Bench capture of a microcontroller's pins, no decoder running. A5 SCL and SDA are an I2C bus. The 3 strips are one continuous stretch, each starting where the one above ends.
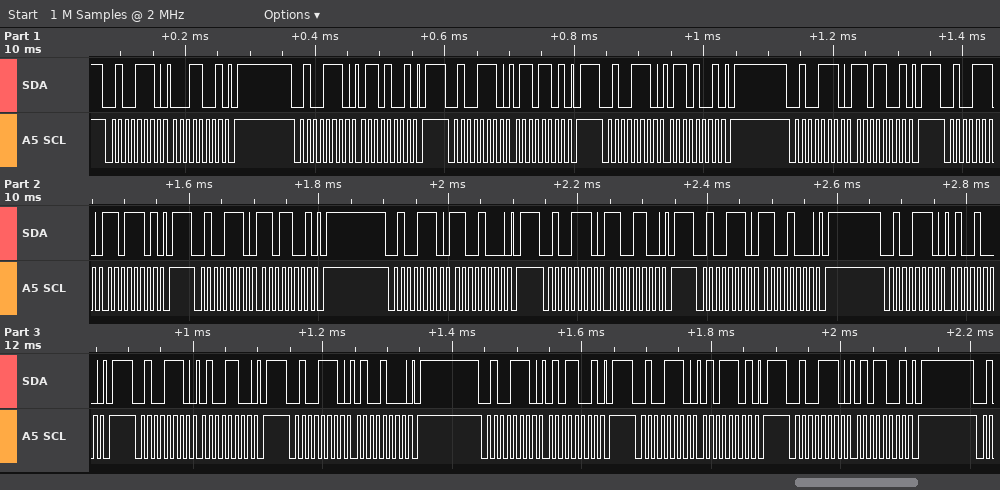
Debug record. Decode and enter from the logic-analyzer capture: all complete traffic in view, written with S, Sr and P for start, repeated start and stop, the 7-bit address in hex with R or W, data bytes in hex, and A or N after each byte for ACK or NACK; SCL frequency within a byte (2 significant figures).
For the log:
S 27W A 19 A P S 27W A 69 A P S 27W A 6D A P S 27W A 69 A P S 27W A D9 A P S 27W A DD A P S 27W A D9 A P S 27W A C8 A P S 27W A CC A P S 27W A C8 A P S 27W A 48 A P S 27W A 4C A P S 27W A 48 A P S 27W A 59 A P S 27W A 5D A P S 27W A 59 A P
100 kHz
